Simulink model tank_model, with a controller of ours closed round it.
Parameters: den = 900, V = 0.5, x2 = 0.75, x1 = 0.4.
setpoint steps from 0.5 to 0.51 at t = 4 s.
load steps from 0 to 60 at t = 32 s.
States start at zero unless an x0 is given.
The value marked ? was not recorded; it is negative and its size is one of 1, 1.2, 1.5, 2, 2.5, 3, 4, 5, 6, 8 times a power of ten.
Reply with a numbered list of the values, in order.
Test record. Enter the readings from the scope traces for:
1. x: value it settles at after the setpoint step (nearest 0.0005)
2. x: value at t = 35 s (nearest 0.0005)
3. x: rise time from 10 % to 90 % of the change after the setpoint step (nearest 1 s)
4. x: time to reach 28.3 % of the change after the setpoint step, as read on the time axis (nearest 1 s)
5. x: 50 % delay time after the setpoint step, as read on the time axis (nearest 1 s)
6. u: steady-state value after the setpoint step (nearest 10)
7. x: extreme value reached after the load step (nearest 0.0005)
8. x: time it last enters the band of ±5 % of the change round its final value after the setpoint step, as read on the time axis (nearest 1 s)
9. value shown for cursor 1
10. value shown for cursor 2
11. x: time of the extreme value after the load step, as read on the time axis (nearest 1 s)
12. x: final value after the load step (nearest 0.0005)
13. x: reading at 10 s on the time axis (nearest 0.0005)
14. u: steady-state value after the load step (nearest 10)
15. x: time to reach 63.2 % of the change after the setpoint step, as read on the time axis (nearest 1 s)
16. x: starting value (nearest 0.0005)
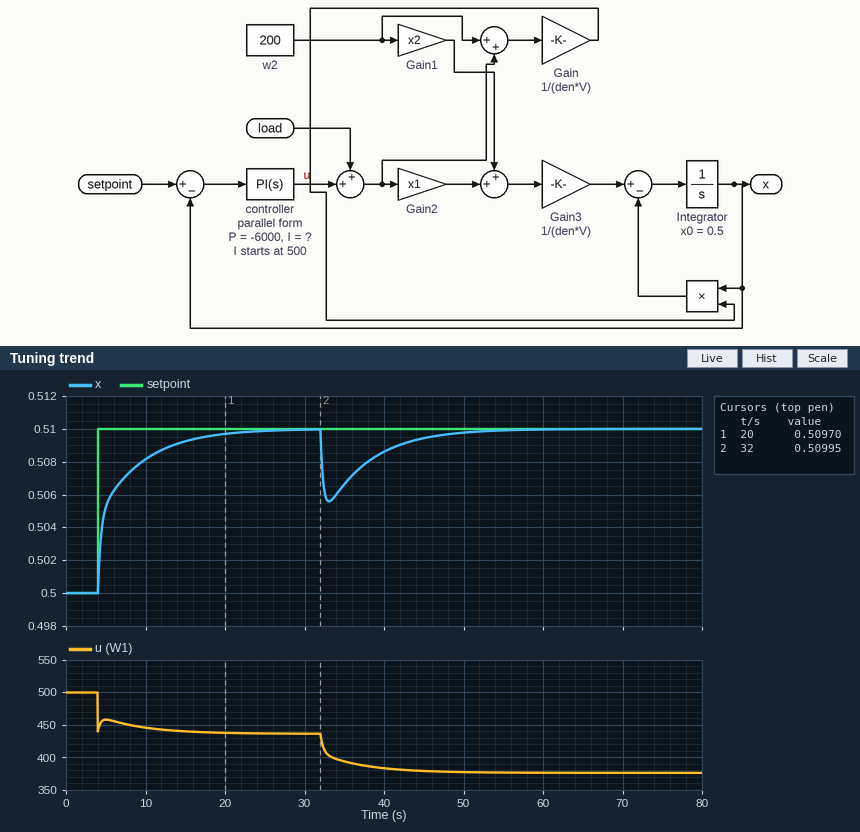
1. 0.5100
2. 0.5065
3. 9 s
4. 4 s
5. 5 s
6. 440
7. 0.5055
8. 17 s
9. 0.50970
10. 0.50995
11. 33 s
12. 0.5100
13. 0.5080
14. 380
15. 6 s
16. 0.5000
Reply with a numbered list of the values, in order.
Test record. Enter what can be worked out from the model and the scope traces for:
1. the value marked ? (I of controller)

1. -2000
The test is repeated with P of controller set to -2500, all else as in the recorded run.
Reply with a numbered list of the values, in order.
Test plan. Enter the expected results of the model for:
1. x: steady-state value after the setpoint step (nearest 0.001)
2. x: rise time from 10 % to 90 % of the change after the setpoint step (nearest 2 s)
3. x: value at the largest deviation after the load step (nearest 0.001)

1. 0.510
2. 8 s
3. 0.504
